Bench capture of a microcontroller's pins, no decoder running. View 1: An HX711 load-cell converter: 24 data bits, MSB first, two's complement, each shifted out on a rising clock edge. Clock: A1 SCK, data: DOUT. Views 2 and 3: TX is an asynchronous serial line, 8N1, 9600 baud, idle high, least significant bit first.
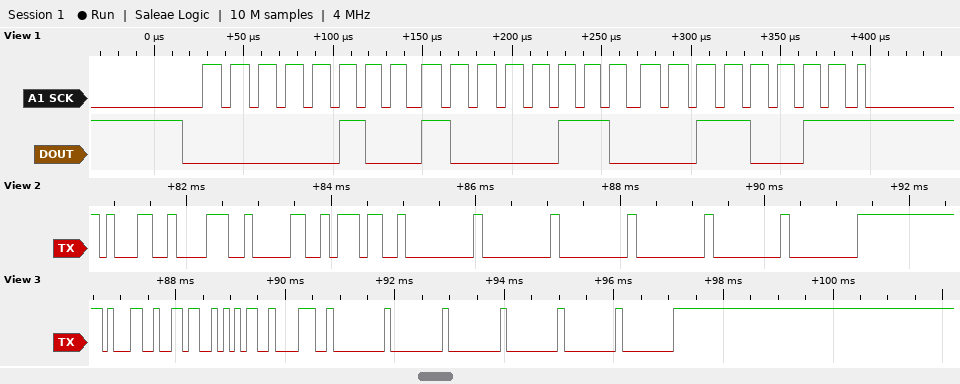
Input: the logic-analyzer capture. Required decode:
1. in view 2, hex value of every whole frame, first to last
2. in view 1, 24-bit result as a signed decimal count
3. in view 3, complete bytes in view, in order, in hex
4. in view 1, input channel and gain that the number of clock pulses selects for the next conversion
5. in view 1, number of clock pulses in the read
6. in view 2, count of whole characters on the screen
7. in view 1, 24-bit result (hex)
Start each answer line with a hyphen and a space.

- 31 38 30 37 00 00 00 00 00 00
- 296499
- 0x31 0x36 0x35 0x38 0x00 0x00 0x00 0x00 0x00 0x00
- channel A, gain 128
- 25
- 10
- 0x048633
